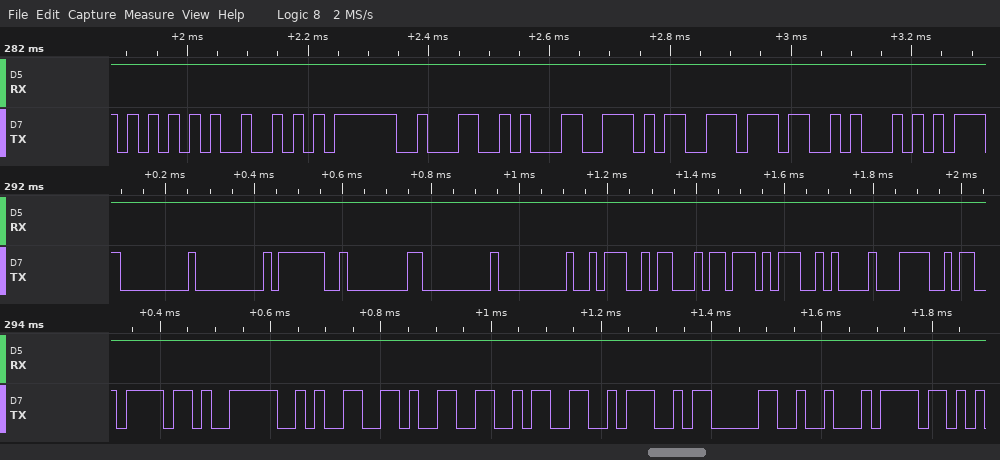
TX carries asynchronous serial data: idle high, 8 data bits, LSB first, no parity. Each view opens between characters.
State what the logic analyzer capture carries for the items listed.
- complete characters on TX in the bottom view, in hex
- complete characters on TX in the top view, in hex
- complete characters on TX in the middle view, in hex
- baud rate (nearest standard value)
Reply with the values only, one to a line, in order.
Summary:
6F, 3E, 99, 99, 9A, 3A, 83, 12, 6F
55, 52, 3F, 4C, CC, CD, 37, 51
00, 00, 3F, 80, 00, 00, 3A, A3, D7, 0A, 3C
57600 baud
